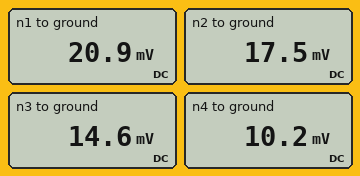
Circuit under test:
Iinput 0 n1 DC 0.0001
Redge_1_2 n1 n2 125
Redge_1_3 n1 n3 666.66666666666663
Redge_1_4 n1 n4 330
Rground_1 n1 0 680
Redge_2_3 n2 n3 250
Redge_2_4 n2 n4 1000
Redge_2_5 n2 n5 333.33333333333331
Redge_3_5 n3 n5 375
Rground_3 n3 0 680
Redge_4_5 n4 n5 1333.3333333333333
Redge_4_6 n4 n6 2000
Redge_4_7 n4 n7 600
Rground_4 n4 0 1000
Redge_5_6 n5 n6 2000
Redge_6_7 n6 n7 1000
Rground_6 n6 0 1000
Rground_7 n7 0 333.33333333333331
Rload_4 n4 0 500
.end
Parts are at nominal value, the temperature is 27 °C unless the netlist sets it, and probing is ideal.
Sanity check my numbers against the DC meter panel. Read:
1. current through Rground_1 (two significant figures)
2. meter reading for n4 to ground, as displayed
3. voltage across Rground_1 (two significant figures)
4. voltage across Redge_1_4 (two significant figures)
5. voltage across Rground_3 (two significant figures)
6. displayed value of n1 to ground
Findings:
31 µA
10.2 mV
21 mV
11 mV
15 mV
20.9 mV
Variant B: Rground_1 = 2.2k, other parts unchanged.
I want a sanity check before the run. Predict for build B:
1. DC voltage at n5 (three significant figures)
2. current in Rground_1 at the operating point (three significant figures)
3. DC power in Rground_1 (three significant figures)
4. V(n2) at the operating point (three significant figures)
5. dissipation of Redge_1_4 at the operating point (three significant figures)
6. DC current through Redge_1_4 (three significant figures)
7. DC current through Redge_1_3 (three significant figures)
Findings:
18.7 mV
12.1 µA
320 nW
22.2 mV
562 nW
41.3 µA
12.0 µA
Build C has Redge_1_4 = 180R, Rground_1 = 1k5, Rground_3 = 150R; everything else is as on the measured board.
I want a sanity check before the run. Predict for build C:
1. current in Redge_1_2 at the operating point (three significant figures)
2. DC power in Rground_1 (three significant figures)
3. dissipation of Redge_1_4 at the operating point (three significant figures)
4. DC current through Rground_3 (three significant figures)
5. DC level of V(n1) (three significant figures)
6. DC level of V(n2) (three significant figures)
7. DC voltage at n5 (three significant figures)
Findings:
34.6 µA
186 nW
277 nW
44.7 µA
16.7 mV
12.4 mV
9.32 mV
